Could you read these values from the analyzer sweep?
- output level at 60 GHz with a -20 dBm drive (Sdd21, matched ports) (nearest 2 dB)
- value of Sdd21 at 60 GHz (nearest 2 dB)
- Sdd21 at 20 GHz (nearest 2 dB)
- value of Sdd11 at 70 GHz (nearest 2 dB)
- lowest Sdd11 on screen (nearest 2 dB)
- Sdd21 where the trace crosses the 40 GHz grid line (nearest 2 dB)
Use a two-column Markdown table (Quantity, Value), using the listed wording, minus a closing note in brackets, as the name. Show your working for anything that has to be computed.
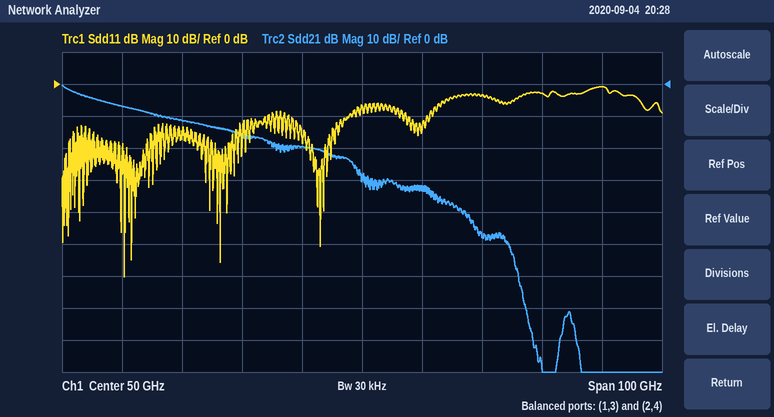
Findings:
| Quantity | Value |
|---|---|
| output level at 60 GHz with a -20 dBm drive (Sdd21, matched ports) | -20 dBm + (-32 dB) = -52 dBm |
| value of Sdd21 at 60 GHz | -32 dB |
| Sdd21 at 20 GHz | -12 dB |
| value of Sdd11 at 70 GHz | -4 dB |
| lowest Sdd11 on screen | -60 dB |
| Sdd21 where the trace crosses the 40 GHz grid line | -20 dB |
